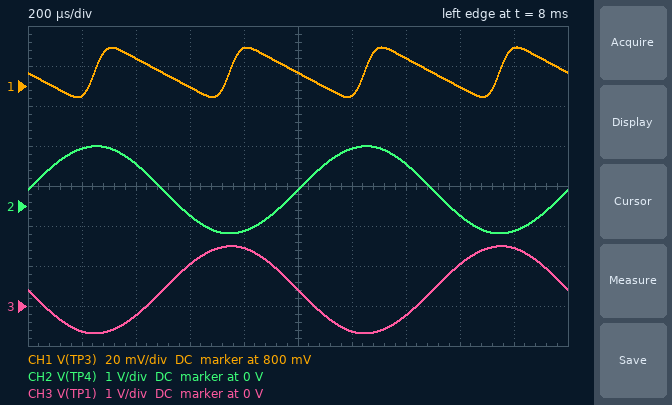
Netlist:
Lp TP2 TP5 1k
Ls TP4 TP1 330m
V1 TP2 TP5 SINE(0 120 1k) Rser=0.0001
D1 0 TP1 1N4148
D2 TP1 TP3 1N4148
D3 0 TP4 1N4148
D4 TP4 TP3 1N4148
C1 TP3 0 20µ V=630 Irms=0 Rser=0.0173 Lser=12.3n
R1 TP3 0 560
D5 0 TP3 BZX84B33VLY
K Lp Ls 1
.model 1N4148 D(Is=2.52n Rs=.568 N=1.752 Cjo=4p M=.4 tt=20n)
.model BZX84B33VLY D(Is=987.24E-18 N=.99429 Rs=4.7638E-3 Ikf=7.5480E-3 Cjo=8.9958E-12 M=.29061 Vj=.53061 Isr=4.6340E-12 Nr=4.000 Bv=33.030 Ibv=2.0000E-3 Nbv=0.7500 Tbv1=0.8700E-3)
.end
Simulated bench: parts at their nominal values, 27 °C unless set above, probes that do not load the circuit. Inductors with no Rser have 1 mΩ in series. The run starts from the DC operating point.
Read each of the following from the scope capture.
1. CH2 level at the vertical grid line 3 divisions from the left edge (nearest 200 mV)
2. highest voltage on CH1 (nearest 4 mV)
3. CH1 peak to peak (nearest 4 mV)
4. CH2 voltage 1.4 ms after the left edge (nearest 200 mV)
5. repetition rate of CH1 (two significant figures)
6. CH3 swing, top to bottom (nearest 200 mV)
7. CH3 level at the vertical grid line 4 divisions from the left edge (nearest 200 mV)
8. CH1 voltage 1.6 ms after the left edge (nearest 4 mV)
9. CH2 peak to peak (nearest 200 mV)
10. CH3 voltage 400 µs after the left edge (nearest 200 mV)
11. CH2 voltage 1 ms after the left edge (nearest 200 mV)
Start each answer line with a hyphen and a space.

- -200 mV
- 820 mV
- 24 mV
- 1.0 V
- 2.0 kHz
- 2.2 V
- 1.4 V
- 800 mV
- 2.2 V
- -200 mV
- 400 mV
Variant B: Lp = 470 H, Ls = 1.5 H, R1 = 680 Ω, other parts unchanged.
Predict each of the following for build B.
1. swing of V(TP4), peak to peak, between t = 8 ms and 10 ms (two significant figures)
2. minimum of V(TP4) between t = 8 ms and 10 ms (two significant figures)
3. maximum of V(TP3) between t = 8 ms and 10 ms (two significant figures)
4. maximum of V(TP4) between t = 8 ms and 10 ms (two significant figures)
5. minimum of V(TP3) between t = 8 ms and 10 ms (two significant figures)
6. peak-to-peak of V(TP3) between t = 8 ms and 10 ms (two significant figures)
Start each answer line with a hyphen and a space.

- 6.8 V
- -810 mV
- 5.2 V
- 6.0 V
- 5.1 V
- 150 mV
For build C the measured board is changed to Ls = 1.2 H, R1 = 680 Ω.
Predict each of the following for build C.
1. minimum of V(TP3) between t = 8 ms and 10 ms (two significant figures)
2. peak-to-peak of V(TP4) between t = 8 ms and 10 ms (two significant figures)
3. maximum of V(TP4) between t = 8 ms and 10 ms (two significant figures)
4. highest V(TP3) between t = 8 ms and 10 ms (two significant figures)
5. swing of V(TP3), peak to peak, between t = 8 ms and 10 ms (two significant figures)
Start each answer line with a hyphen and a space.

- 2.6 V
- 4.2 V
- 3.4 V
- 2.7 V
- 73 mV
